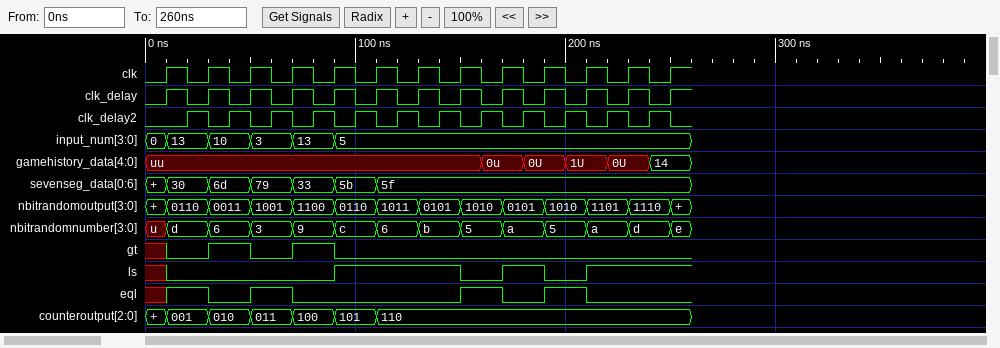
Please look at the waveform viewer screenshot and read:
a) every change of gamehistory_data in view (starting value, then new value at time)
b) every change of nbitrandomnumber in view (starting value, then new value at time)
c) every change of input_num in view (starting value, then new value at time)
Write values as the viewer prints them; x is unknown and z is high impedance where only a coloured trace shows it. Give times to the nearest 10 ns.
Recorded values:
uu, 0u at 160 ns, 0U at 180 ns, 1U at 200 ns, 0U at 220 ns, 14 at 240 ns
u, d at 10 ns, 6 at 30 ns, 3 at 50 ns, 9 at 70 ns, c at 90 ns, 6 at 110 ns, b at 130 ns, 5 at 150 ns, a at 170 ns, 5 at 190 ns, a at 210 ns, d at 230 ns, e at 250 ns
0, 13 at 10 ns, 10 at 30 ns, 3 at 50 ns, 13 at 70 ns, 5 at 90 ns
